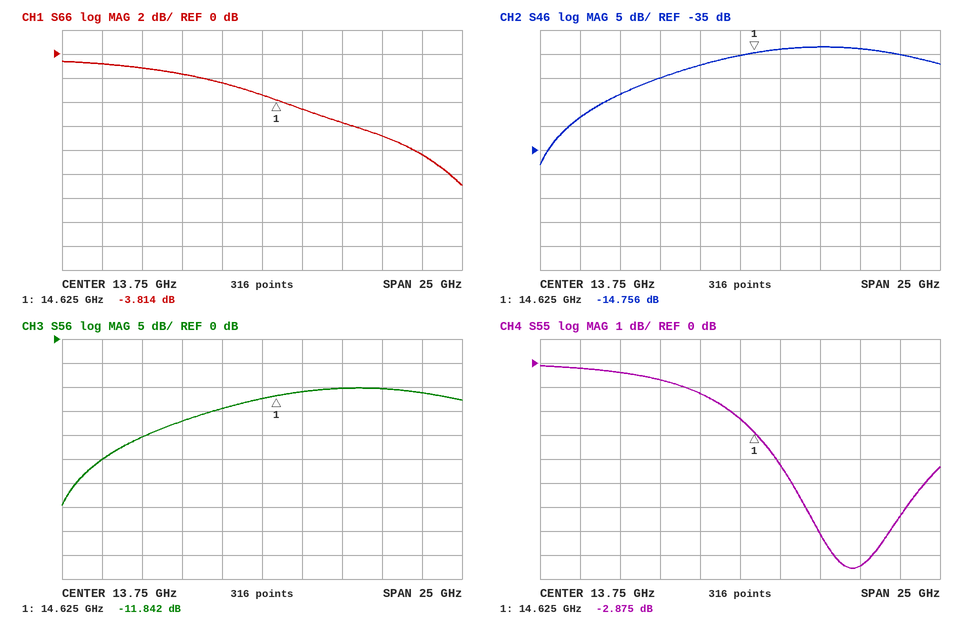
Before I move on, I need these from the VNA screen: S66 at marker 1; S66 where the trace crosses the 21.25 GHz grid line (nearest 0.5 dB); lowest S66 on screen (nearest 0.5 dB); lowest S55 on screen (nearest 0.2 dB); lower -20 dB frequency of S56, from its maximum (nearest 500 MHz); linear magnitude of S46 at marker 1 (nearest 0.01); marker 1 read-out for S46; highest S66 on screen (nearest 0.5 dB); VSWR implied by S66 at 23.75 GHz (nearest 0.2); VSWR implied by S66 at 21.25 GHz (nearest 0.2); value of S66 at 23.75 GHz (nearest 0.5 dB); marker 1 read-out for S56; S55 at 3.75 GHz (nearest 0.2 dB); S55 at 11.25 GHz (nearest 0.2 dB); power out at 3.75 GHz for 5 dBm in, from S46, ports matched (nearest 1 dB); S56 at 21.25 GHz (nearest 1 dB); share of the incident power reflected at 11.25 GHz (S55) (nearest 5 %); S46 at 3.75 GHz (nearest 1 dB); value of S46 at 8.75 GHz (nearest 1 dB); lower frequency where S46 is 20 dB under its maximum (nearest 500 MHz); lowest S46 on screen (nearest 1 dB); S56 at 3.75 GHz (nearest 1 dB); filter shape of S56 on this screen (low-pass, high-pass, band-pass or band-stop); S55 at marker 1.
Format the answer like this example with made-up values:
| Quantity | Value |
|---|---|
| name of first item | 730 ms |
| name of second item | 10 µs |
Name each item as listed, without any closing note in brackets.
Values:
| Quantity | Value |
|---|---|
| S66 at marker 1 | -3.814 dB |
| S66 where the trace crosses the 21.25 GHz grid line | -7.0 dB |
| lowest S66 on screen | -11.0 dB |
| lowest S55 on screen | -8.6 dB |
| lower -20 dB frequency of S56, from its maximum | 2.0 GHz |
| linear magnitude of S46 at marker 1 | 0.18 |
| marker 1 read-out for S46 | -14.756 dB |
| highest S66 on screen | -0.5 dB |
| VSWR implied by S66 at 23.75 GHz | 2.2 |
| VSWR implied by S66 at 21.25 GHz | 2.6 |
| value of S66 at 23.75 GHz | -8.5 dB |
| marker 1 read-out for S56 | -11.842 dB |
| S55 at 3.75 GHz | -0.2 dB |
| S55 at 11.25 GHz | -1.2 dB |
| power out at 3.75 GHz for 5 dBm in, from S46, ports matched | -23 dBm |
| S56 at 21.25 GHz | -10 dB |
| share of the incident power reflected at 11.25 GHz (S55) | 75 % |
| S46 at 3.75 GHz | -28 dB |
| value of S46 at 8.75 GHz | -20 dB |
| lower frequency where S46 is 20 dB under its maximum | 2.0 GHz |
| lowest S46 on screen | -38 dB |
| S56 at 3.75 GHz | -25 dB |
| filter shape of S56 on this screen | high-pass |
| S55 at marker 1 | -2.875 dB |
